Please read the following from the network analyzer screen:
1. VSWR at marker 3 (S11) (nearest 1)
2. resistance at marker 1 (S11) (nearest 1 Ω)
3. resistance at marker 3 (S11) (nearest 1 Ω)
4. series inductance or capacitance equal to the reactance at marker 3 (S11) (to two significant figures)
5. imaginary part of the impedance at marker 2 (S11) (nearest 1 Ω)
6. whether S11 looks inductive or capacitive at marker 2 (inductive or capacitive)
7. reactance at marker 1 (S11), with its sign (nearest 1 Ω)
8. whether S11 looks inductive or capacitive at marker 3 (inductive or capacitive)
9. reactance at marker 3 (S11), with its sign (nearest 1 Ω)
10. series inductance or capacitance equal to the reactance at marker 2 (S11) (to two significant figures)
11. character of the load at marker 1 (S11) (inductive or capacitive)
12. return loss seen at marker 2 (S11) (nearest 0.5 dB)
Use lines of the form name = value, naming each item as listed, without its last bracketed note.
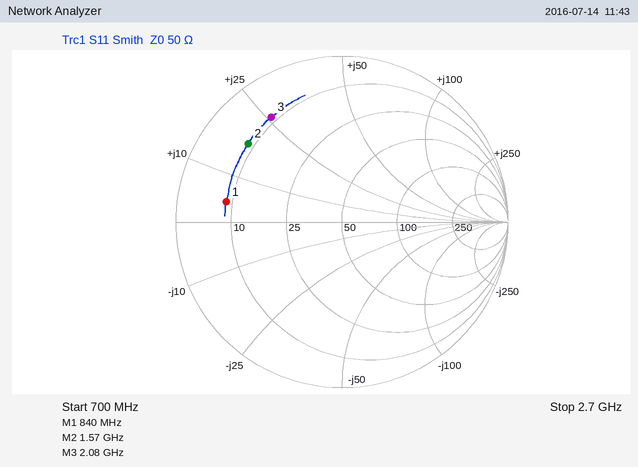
VSWR at marker 3 (S11) = 7
resistance at marker 1 (S11) = 9 Ω
resistance at marker 3 (S11) = 9 Ω
series inductance or capacitance equal to the reactance at marker 3 (S11) = 2.0 nH
imaginary part of the impedance at marker 2 (S11) = +18 Ω
whether S11 looks inductive or capacitive at marker 2 = inductive
reactance at marker 1 (S11), with its sign = +4 Ω
whether S11 looks inductive or capacitive at marker 3 = inductive
reactance at marker 3 (S11), with its sign = +26 Ω
series inductance or capacitance equal to the reactance at marker 2 (S11) = 1.8 nH
character of the load at marker 1 (S11) = inductive
return loss seen at marker 2 (S11) = 2.5 dB
